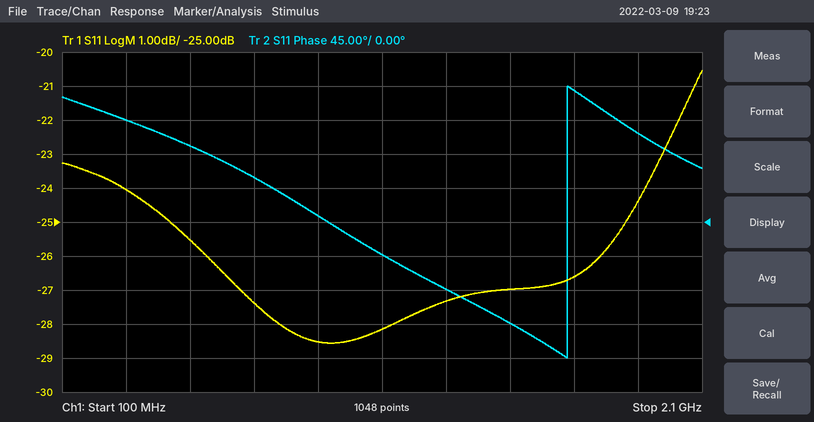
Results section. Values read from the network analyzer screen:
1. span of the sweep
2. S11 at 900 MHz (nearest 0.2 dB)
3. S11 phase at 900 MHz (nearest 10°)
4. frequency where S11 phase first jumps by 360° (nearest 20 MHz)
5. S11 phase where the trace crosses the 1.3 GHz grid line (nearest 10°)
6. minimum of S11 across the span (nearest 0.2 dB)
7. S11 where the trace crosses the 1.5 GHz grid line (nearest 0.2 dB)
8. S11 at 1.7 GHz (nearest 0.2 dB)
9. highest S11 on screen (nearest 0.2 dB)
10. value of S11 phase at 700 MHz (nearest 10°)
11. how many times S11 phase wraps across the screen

2 GHz
-28.6 dB
10°
1.68 GHz
-90°
-28.6 dB
-27.0 dB
-26.6 dB
-20.6 dB
60°
1
